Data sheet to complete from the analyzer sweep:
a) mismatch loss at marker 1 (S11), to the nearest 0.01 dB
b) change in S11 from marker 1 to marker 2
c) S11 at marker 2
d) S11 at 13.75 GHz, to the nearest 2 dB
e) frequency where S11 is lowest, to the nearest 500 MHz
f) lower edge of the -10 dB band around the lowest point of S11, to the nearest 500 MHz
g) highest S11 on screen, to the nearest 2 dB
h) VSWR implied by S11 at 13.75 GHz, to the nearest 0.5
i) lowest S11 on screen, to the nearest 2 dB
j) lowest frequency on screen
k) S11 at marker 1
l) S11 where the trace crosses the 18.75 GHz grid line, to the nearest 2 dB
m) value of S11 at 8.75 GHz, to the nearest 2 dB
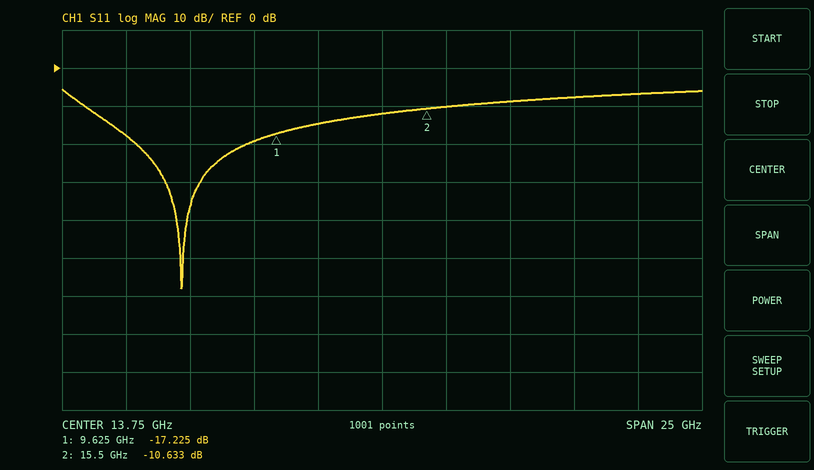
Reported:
0.08 dB
6.592 dB
-10.633 dB
-12 dB
6.0 GHz
2.0 GHz
-6 dB
1.5
-58 dB
1.25 GHz
-17.225 dB
-8 dB
-20 dB
